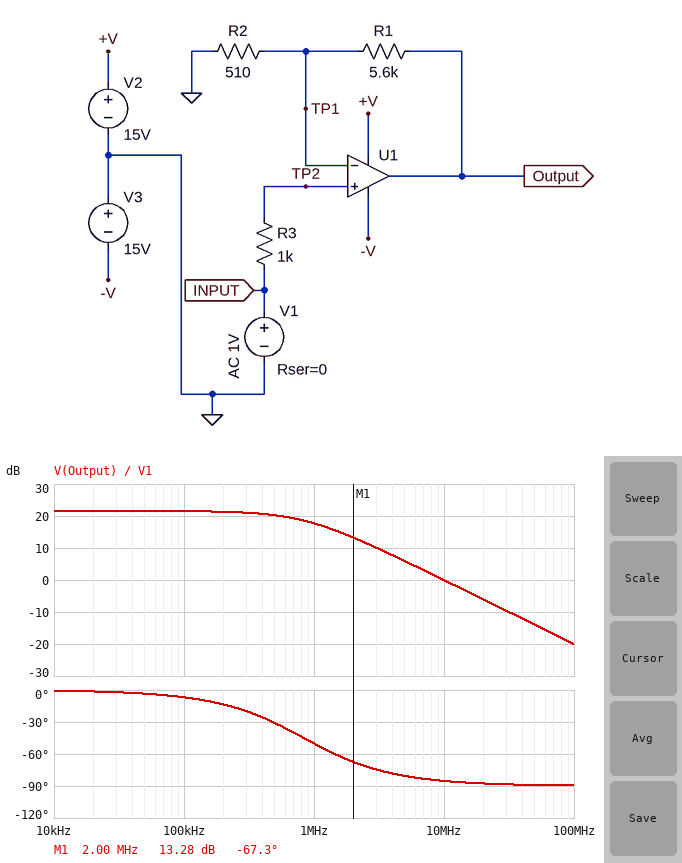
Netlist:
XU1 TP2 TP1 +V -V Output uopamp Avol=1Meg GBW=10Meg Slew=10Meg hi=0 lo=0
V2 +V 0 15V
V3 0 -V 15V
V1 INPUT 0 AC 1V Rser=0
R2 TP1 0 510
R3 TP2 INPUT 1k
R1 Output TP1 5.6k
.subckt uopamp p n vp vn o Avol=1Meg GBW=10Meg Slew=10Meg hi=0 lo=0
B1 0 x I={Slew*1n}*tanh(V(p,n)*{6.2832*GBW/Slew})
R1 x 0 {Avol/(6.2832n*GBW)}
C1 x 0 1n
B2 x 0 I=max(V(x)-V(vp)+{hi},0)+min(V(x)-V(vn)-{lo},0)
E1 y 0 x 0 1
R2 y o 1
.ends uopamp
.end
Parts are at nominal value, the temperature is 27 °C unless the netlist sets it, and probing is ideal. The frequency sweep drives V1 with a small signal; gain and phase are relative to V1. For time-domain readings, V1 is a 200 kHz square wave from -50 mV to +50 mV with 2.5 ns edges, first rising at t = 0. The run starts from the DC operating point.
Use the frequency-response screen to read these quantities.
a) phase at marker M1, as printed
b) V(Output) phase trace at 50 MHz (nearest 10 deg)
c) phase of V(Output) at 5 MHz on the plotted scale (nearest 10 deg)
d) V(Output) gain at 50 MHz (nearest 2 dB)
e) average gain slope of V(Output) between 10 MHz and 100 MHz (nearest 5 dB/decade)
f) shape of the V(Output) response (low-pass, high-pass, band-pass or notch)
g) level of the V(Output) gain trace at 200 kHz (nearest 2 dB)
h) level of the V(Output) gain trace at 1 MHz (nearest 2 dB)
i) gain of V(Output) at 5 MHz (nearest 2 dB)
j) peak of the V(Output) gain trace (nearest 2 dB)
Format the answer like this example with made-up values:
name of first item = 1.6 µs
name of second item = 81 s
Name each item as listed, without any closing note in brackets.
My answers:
phase at marker M1, as printed = -67.3 deg
V(Output) phase trace at 50 MHz = -90 deg
phase of V(Output) at 5 MHz on the plotted scale = -80 deg
V(Output) gain at 50 MHz = -14 dB
average gain slope of V(Output) between 10 MHz and 100 MHz = -20 dB/decade
shape of the V(Output) response = low-pass
level of the V(Output) gain trace at 200 kHz = 22 dB
level of the V(Output) gain trace at 1 MHz = 18 dB
gain of V(Output) at 5 MHz = 6 dB
peak of the V(Output) gain trace = 22 dB
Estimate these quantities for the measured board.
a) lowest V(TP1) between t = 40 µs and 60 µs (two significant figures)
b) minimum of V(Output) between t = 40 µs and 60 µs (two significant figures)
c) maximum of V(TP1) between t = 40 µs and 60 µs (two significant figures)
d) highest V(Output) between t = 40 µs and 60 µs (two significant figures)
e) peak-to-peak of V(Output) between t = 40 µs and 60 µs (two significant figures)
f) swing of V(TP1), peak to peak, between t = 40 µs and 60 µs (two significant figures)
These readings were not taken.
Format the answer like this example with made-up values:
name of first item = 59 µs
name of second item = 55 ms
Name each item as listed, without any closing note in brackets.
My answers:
lowest V(TP1) between t = 40 µs and 60 µs = -50 mV
minimum of V(Output) between t = 40 µs and 60 µs = -600 mV
maximum of V(TP1) between t = 40 µs and 60 µs = 50 mV
highest V(Output) between t = 40 µs and 60 µs = 600 mV
peak-to-peak of V(Output) between t = 40 µs and 60 µs = 1.2 V
swing of V(TP1), peak to peak, between t = 40 µs and 60 µs = 100 mV
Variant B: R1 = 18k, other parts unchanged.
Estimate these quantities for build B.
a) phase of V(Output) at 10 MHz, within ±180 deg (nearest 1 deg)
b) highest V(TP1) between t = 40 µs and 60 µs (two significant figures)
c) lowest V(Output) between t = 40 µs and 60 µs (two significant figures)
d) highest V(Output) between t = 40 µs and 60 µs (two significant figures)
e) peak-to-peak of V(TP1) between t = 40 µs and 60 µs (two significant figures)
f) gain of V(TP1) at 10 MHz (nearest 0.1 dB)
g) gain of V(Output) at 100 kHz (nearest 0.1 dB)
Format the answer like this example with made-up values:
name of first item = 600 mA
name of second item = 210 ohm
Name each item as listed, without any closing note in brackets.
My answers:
phase of V(Output) at 10 MHz, within ±180 deg = -88 deg
highest V(TP1) between t = 40 µs and 60 µs = 49 mV
lowest V(Output) between t = 40 µs and 60 µs = -1.8 V
highest V(Output) between t = 40 µs and 60 µs = 1.8 V
peak-to-peak of V(TP1) between t = 40 µs and 60 µs = 97 mV
gain of V(TP1) at 10 MHz = -31.2 dB
gain of V(Output) at 100 kHz = 30.7 dB
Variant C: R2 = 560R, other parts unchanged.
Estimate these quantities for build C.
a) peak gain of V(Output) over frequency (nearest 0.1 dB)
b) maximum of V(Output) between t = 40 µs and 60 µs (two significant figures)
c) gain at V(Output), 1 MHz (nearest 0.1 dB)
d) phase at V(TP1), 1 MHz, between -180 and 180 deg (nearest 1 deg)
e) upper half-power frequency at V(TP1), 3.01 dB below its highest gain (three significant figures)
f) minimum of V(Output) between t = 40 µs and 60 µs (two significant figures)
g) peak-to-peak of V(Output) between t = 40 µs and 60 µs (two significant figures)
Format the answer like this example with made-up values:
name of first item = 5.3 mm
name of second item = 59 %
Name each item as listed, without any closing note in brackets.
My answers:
peak gain of V(Output) over frequency = 20.8 dB
maximum of V(Output) between t = 40 µs and 60 µs = 550 mV
gain at V(Output), 1 MHz = 17.4 dB
phase at V(TP1), 1 MHz, between -180 and 180 deg = -48 deg
upper half-power frequency at V(TP1), 3.01 dB below its highest gain = 909 kHz
minimum of V(Output) between t = 40 µs and 60 µs = -550 mV
peak-to-peak of V(Output) between t = 40 µs and 60 µs = 1.1 V
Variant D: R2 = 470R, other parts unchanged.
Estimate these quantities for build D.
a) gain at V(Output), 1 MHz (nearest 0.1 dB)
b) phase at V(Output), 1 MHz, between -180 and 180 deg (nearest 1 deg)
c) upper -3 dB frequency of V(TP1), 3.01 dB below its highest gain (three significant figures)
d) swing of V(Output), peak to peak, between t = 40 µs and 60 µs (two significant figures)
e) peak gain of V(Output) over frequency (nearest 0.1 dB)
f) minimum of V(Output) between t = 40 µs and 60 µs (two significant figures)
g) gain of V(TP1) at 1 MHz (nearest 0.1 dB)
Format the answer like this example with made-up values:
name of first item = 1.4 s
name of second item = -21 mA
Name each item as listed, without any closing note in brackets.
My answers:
gain at V(Output), 1 MHz = 18.0 dB
phase at V(Output), 1 MHz, between -180 and 180 deg = -52 deg
upper -3 dB frequency of V(TP1), 3.01 dB below its highest gain = 774 kHz
swing of V(Output), peak to peak, between t = 40 µs and 60 µs = 1.3 V
peak gain of V(Output) over frequency = 22.2 dB
minimum of V(Output) between t = 40 µs and 60 µs = -650 mV
gain of V(TP1) at 1 MHz = -4.3 dB
